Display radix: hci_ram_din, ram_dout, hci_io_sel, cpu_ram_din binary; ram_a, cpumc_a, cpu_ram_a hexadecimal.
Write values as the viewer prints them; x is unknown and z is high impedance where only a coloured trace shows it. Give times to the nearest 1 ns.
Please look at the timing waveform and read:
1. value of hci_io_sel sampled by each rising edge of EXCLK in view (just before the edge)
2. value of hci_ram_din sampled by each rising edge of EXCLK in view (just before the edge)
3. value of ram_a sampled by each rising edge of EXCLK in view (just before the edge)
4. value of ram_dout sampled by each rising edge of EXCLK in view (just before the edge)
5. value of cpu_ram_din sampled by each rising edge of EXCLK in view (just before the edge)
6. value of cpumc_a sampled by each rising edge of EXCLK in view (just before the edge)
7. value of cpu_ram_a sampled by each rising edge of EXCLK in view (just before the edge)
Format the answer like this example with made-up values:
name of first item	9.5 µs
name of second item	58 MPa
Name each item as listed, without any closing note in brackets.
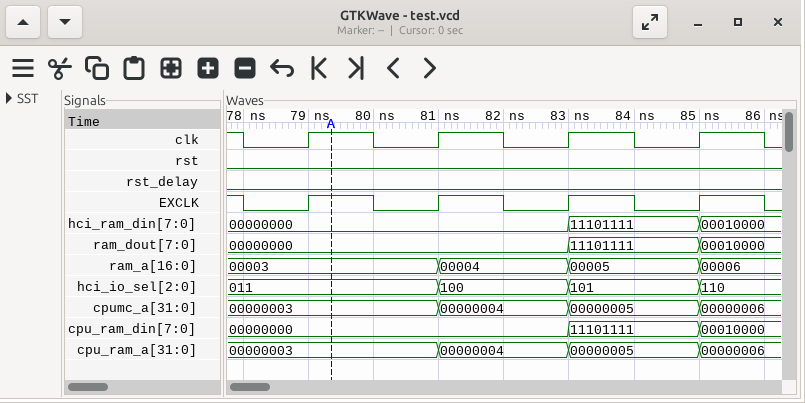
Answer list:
value of hci_io_sel sampled by each rising edge of EXCLK in view	011, 011, 100, 101
value of hci_ram_din sampled by each rising edge of EXCLK in view	00000000, 00000000, 00000000, 11101111
value of ram_a sampled by each rising edge of EXCLK in view	00003, 00003, 00004, 00005
value of ram_dout sampled by each rising edge of EXCLK in view	00000000, 00000000, 00000000, 11101111
value of cpu_ram_din sampled by each rising edge of EXCLK in view	00000000, 00000000, 00000000, 11101111
value of cpumc_a sampled by each rising edge of EXCLK in view	00000003, 00000003, 00000004, 00000005
value of cpu_ram_a sampled by each rising edge of EXCLK in view	00000003, 00000003, 00000004, 00000005
